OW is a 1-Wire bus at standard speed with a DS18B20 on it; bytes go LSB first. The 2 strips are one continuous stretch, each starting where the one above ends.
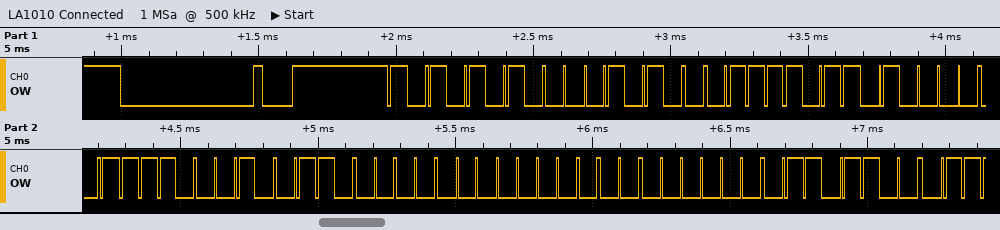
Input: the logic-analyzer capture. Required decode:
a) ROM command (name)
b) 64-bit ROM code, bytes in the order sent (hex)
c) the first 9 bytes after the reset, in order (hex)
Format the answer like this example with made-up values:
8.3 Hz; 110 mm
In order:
Match ROM; 28 DE 82 47 06 00 00 36; 55 28 DE 82 47 06 00 00 36
